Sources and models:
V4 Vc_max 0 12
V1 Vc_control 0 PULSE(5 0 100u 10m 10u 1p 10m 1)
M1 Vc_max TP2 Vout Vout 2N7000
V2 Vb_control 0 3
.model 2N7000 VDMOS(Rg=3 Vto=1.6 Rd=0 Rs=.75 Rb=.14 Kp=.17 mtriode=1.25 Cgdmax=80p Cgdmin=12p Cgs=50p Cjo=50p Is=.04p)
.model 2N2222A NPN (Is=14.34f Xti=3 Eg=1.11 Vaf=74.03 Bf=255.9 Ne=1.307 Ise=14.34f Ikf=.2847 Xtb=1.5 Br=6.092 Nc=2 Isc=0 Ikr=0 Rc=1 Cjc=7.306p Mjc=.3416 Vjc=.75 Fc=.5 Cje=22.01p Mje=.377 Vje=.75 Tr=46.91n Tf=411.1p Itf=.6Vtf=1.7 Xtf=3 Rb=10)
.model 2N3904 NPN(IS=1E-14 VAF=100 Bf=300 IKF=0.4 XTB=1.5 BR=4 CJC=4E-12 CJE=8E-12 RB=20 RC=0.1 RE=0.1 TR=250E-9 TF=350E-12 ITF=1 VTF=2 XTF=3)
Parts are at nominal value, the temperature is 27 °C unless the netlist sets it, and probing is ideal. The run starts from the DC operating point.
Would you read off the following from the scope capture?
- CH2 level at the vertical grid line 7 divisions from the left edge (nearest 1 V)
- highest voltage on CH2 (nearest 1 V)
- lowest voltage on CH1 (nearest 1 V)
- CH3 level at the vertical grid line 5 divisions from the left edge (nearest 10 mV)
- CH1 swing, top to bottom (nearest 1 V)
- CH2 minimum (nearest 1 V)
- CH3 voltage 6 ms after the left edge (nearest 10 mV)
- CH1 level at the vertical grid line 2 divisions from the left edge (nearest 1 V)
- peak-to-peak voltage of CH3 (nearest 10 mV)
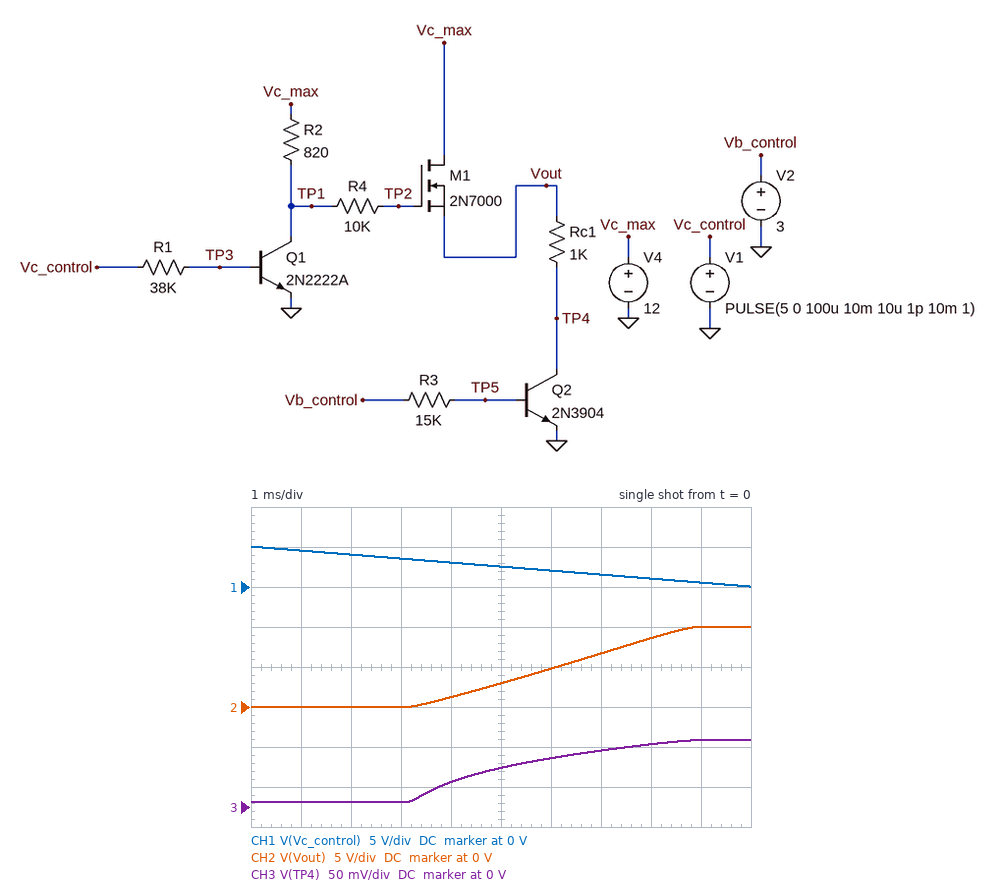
7 V
10 V
0 V
50 mV
5 V
0 V
60 mV
4 V
80 mV
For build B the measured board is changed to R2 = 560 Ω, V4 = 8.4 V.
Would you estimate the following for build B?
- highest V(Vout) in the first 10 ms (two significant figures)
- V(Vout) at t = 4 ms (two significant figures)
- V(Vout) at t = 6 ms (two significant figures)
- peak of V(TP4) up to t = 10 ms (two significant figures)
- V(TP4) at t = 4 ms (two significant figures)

6.5 V
620 mV
3.0 V
70 mV
21 mV
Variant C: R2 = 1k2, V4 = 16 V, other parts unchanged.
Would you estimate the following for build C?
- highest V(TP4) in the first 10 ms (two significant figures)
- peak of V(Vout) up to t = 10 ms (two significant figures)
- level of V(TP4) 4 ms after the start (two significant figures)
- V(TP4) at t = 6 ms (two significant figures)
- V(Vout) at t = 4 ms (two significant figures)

96 mV
14 V
29 mV
68 mV
1.1 V
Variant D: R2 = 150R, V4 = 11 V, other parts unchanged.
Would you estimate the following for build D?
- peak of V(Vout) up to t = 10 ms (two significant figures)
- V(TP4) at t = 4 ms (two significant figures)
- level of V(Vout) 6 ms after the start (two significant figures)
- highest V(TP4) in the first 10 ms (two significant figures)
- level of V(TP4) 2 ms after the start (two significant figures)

9.1 V
73 mV
8.1 V
80 mV
70 mV
